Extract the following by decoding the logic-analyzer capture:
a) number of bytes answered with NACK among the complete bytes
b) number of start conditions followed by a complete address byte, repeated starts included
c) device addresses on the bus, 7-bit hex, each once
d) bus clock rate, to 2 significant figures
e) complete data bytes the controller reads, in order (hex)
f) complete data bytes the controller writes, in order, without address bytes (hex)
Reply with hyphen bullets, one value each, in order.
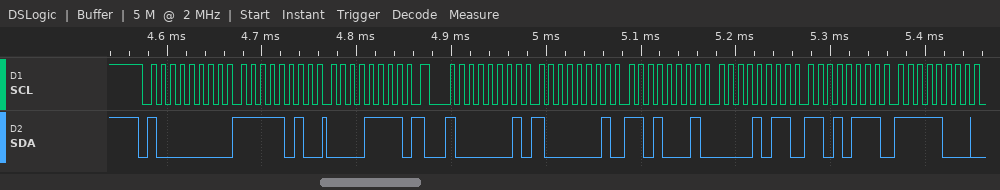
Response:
- 0
- 2
- 0x40
- 100 kHz
- 81 D1 0B D7 F8
- FA 0F
